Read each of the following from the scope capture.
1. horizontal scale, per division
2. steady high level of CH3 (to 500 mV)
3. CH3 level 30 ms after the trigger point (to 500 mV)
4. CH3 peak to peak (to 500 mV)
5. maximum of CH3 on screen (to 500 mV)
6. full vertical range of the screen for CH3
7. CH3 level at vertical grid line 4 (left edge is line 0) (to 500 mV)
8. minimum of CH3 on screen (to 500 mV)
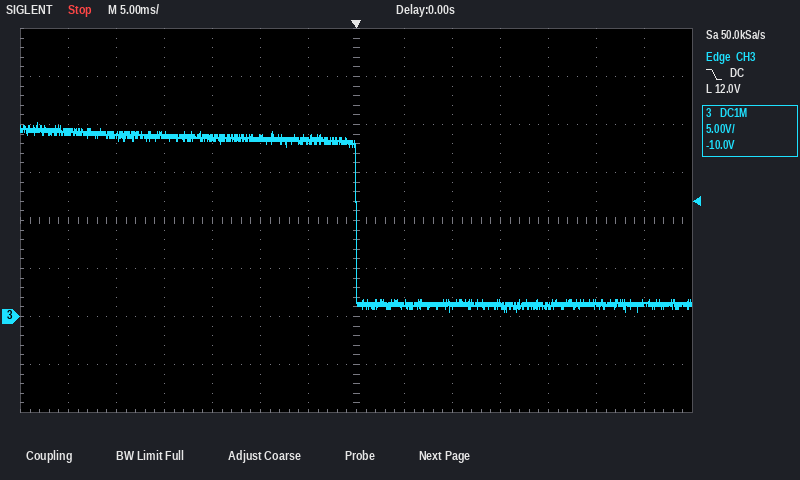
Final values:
5 ms
18.5 V
1.5 V
19.5 V
20.0 V
40 V
18.5 V
500 mV
